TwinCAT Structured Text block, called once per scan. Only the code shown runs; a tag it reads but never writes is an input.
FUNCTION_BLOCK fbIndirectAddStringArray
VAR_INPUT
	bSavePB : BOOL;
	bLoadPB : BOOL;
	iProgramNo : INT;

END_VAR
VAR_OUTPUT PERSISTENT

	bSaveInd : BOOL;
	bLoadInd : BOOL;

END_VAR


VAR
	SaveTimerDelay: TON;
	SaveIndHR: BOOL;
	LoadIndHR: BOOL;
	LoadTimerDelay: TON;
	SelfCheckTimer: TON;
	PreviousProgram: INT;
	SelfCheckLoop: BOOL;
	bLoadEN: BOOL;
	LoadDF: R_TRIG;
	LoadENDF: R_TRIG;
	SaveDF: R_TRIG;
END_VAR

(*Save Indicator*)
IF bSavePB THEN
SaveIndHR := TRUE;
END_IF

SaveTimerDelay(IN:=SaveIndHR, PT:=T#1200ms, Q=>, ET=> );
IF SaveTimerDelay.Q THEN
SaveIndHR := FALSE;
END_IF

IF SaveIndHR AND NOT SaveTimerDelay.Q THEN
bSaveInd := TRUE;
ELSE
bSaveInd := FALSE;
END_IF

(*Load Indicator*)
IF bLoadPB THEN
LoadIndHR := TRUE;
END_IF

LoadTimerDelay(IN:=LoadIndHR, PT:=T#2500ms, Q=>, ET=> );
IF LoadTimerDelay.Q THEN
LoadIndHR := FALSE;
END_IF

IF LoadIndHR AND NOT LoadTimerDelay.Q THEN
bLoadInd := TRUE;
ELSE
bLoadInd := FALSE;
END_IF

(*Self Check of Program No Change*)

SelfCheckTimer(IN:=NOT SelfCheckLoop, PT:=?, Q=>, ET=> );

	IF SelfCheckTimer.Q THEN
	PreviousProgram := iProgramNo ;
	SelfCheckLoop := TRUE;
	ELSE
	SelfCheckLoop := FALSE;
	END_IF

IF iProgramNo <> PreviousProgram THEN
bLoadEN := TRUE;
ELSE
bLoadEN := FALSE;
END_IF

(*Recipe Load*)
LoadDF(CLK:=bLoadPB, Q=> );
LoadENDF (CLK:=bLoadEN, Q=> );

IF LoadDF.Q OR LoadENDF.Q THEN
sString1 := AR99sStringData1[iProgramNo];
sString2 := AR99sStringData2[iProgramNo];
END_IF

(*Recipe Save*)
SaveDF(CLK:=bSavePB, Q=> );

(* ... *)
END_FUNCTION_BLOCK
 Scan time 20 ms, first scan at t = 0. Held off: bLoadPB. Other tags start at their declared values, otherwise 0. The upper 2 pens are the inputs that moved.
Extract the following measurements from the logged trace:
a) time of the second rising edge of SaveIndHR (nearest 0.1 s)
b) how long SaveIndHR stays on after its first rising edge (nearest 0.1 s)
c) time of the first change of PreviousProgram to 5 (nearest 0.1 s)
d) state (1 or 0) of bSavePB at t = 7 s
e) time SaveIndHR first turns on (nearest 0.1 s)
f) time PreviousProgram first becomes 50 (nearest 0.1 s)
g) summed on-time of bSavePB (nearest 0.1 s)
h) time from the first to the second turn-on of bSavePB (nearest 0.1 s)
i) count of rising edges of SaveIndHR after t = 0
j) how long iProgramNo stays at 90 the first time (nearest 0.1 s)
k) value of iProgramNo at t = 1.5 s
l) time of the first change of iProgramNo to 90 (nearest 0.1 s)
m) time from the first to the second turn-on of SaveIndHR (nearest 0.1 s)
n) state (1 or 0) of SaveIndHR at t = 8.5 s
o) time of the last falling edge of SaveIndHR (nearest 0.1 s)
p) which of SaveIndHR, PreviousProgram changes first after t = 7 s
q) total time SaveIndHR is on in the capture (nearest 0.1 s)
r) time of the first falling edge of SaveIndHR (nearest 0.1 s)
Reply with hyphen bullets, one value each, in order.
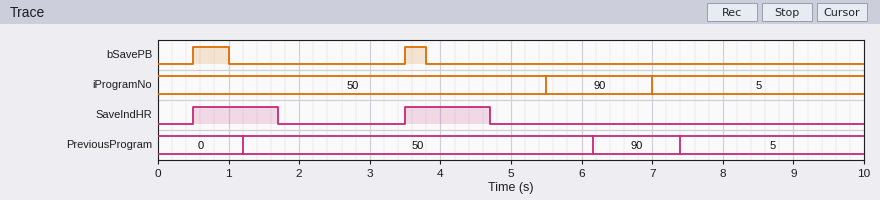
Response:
- 3.5 s
- 1.2 s
- 7.4 s
- 0
- 0.5 s
- 1.2 s
- 0.8 s
- 3.0 s
- 2
- 1.5 s
- 50
- 5.5 s
- 3.0 s
- 0
- 4.7 s
- PreviousProgram
- 2.4 s
- 1.7 s
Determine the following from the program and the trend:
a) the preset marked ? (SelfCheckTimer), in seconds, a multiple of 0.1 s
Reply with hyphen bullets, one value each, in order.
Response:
- 1.2 s
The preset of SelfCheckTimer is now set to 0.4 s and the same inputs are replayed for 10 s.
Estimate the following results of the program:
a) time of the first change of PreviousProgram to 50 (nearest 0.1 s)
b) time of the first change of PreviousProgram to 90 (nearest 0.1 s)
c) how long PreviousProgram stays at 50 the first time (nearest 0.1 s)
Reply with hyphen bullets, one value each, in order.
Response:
- 0.4 s
- 5.7 s
- 5.3 s
